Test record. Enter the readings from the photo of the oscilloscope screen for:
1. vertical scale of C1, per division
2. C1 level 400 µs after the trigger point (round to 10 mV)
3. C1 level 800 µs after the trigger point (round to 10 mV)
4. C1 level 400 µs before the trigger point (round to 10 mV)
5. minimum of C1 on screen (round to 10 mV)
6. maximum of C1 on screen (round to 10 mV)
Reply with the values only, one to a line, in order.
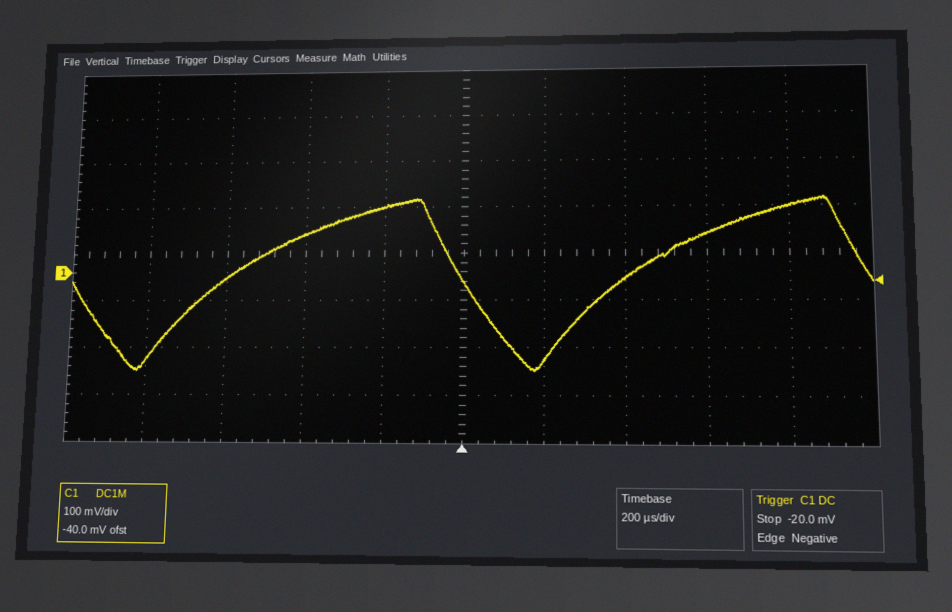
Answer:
100 mV
-10 mV
140 mV
80 mV
-210 mV
160 mV
